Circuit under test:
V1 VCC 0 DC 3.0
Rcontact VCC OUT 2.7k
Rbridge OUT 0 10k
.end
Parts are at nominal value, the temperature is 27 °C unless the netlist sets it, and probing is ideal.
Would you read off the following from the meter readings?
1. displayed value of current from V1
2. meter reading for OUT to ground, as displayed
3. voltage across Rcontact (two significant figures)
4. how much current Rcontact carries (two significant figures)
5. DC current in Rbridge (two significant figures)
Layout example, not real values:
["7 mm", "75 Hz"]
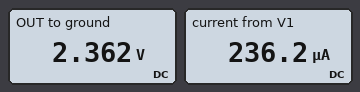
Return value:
["236.2 µA", "2.362 V", "640 mV", "240 µA", "240 µA"]
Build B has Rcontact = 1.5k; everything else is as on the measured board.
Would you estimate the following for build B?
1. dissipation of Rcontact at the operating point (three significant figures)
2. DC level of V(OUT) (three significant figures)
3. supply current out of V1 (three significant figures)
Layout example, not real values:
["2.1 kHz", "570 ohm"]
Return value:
["102 µW", "2.61 V", "261 µA"]
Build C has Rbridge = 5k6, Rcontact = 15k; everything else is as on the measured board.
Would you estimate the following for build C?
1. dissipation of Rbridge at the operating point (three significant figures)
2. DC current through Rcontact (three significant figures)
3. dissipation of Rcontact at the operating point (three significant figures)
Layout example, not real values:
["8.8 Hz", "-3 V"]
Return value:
["119 µW", "146 µA", "318 µW"]
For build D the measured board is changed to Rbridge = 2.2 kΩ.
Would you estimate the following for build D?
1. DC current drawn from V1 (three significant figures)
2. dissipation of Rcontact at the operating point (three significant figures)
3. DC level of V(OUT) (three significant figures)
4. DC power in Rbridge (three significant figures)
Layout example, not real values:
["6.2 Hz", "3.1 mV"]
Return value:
["612 µA", "1.01 mW", "1.35 V", "825 µW"]
